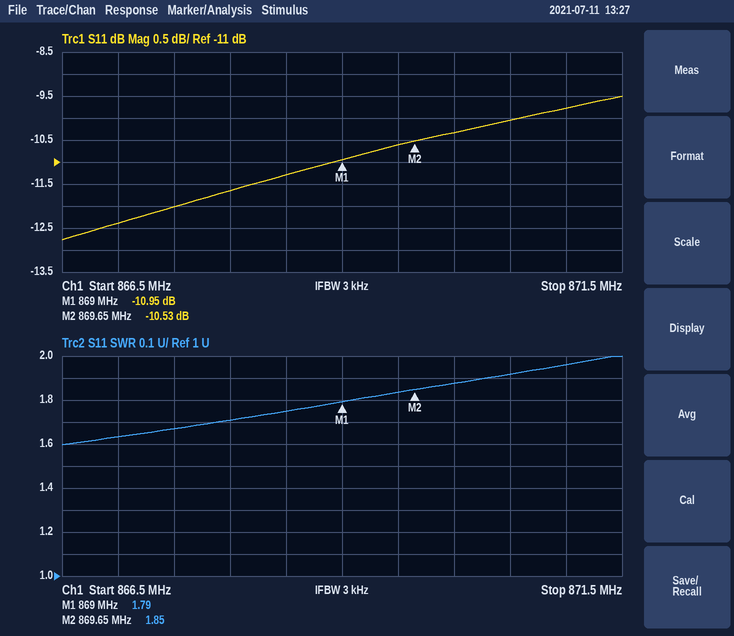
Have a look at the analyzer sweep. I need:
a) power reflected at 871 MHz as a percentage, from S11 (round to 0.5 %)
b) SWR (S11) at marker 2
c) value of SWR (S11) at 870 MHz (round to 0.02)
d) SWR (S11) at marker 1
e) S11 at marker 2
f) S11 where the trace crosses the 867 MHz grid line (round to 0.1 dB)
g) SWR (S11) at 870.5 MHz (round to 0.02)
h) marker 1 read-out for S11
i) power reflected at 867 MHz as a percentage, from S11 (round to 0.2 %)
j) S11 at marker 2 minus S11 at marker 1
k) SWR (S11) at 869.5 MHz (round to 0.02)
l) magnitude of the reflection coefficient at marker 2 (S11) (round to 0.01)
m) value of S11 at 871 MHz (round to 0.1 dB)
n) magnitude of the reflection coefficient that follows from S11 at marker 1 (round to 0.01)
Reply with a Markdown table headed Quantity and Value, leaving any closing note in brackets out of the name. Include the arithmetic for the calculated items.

| Quantity | Value |
|---|---|
| power reflected at 871 MHz as a percentage, from S11 | 10^(-9.8/10) ≈ 10.5 % |
| SWR (S11) at marker 2 | 1.85 |
| value of SWR (S11) at 870 MHz | 1.88 |
| SWR (S11) at marker 1 | 1.79 |
| S11 at marker 2 | -10.53 dB |
| S11 where the trace crosses the 867 MHz grid line | -12.4 dB |
| SWR (S11) at 870.5 MHz | 1.92 |
| marker 1 read-out for S11 | -10.95 dB |
| power reflected at 867 MHz as a percentage, from S11 | 10^(-12.4/10) ≈ 5.8 % |
| S11 at marker 2 minus S11 at marker 1 | -10.53 − (-10.95) = 0.42 dB |
| SWR (S11) at 869.5 MHz | 1.84 |
| magnitude of the reflection coefficient at marker 2 (S11) | 10^(-10.53/20) ≈ 0.30 |
| value of S11 at 871 MHz | -9.8 dB |
| magnitude of the reflection coefficient that follows from S11 at marker 1 | 10^(-10.95/20) ≈ 0.28 |
